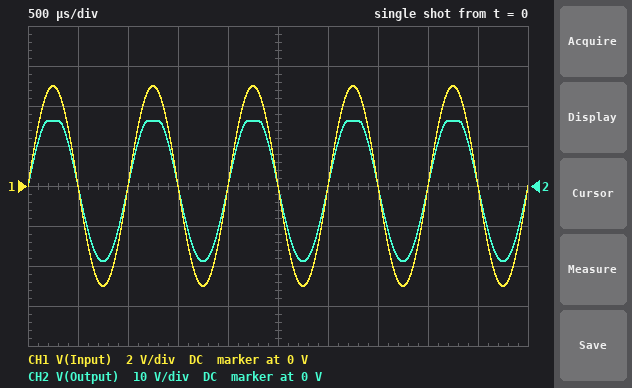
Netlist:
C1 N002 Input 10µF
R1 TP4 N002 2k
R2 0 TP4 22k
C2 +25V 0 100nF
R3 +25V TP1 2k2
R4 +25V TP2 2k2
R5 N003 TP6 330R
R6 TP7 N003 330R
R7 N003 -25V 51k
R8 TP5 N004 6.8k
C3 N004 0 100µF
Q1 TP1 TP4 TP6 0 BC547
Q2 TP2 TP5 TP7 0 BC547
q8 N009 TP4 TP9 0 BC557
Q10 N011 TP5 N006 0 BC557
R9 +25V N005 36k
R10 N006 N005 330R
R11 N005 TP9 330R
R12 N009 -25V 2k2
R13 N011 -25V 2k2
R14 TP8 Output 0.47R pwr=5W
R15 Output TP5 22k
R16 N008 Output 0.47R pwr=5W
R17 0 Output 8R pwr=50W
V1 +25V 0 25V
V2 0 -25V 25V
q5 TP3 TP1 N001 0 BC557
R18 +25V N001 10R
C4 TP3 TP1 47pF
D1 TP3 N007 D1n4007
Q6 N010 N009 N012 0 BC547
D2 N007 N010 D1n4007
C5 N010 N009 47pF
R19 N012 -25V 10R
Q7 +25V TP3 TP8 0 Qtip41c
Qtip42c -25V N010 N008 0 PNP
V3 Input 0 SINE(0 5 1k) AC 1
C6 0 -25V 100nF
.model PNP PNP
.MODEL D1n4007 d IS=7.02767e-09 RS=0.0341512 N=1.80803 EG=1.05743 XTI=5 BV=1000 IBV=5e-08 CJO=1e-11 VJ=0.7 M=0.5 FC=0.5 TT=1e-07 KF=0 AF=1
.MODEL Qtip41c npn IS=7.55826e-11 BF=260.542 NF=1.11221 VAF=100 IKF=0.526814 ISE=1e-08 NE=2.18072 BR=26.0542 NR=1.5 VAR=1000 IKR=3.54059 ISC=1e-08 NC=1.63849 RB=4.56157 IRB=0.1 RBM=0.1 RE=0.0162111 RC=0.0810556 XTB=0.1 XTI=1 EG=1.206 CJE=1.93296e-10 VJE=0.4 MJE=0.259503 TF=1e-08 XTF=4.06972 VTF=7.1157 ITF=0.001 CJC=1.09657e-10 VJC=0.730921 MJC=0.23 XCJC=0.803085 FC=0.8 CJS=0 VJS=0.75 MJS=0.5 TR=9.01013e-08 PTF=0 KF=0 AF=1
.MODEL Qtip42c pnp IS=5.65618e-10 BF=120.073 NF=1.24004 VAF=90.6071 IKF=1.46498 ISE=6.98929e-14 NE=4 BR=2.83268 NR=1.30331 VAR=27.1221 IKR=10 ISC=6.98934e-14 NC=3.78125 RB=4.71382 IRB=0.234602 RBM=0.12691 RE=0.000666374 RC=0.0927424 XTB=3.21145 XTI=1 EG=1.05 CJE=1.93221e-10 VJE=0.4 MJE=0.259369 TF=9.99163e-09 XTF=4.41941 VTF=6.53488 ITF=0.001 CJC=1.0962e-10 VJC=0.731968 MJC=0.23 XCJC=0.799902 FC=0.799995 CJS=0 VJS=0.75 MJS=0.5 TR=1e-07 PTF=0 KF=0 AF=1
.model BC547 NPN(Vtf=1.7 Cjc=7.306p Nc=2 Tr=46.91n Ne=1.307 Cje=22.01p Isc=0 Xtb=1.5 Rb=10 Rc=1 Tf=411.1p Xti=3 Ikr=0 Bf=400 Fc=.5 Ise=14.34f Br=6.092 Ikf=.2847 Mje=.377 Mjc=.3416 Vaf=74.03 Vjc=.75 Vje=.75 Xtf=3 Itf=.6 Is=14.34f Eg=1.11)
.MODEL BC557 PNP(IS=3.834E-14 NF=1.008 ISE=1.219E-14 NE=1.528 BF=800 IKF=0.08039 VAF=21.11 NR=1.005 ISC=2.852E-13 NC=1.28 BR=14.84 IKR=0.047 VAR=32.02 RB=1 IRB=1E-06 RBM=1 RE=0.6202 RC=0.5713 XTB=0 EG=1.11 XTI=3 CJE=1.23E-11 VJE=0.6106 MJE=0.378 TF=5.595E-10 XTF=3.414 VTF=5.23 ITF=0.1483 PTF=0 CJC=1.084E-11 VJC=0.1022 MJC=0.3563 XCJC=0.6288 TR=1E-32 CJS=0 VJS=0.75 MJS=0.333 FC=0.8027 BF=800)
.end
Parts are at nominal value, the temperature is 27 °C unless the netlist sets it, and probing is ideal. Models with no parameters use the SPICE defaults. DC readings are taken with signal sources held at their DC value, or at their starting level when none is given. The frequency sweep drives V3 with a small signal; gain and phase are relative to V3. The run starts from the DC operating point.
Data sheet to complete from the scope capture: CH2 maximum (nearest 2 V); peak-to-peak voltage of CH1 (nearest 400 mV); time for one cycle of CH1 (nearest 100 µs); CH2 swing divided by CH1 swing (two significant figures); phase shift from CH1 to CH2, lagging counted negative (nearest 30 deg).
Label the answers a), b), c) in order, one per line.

a) 16 V
b) 10.0 V
c) 1.0 ms
d) 3.5
e) 0 deg
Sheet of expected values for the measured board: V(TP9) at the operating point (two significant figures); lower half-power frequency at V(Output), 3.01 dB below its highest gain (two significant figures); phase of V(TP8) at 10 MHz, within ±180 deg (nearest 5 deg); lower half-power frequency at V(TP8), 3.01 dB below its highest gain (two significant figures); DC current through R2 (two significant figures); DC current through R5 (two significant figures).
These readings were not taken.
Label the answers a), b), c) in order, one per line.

a) 550 mV
b) 730 mHz
c) 170 deg
d) 730 mHz
e) 1.2 µA
f) 280 µA
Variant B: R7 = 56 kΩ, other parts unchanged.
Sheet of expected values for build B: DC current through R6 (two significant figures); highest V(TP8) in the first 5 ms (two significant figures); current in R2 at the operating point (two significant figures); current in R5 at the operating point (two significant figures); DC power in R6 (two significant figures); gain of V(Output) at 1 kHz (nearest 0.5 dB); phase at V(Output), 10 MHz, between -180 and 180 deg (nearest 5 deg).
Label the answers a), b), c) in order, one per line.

a) 170 µA
b) 16 V
c) 1.1 µA
d) 270 µA
e) 9.3 µW
f) 11.0 dB
g) 155 deg
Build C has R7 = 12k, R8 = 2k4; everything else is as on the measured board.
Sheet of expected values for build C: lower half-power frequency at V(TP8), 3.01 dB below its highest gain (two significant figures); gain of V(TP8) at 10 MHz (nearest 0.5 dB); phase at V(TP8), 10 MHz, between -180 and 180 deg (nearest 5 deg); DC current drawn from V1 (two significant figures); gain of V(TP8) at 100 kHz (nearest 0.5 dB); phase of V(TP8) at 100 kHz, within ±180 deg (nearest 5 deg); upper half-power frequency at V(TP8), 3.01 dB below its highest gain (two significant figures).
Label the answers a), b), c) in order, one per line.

a) 1.0 Hz
b) -24.0 dB
c) -165 deg
d) 110 mA
e) 19.0 dB
f) -20 deg
g) 300 kHz
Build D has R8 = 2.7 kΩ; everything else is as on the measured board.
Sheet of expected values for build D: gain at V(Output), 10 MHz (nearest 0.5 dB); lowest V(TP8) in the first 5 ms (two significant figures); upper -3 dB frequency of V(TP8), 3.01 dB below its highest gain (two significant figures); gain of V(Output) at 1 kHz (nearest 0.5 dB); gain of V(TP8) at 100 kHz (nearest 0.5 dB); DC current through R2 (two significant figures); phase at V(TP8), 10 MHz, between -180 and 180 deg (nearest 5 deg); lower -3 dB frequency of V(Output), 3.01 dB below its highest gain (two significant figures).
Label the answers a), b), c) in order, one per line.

a) -25.0 dB
b) -22 V
c) 270 kHz
d) 17.5 dB
e) 17.0 dB
f) 1.2 µA
g) 165 deg
h) 940 mHz
